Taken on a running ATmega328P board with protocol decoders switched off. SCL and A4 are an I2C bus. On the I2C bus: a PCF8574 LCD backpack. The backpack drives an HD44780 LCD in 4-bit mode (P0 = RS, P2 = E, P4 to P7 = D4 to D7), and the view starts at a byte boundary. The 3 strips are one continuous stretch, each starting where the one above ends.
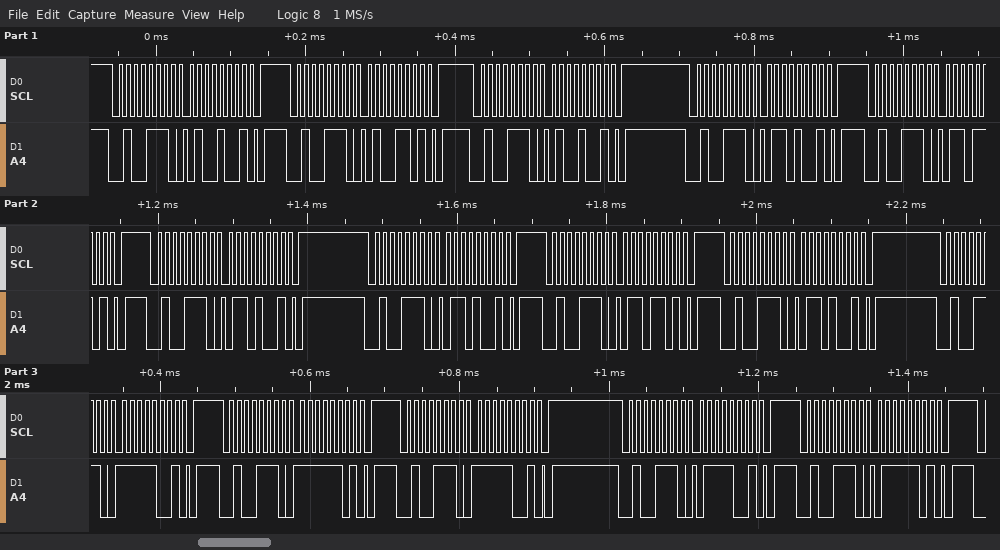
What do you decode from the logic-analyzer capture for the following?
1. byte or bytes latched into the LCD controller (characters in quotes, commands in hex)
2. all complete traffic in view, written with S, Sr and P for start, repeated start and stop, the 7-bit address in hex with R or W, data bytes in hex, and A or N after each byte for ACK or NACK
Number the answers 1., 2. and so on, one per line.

1. 'F' 'o'
2. S 27W A 49 A P S 27W A 4D A P S 27W A 49 A P S 27W A 69 A P S 27W A 6D A P S 27W A 69 A P S 27W A 69 A P S 27W A 6D A P S 27W A 69 A P S 27W A F9 A P S 27W A FD A P S 27W A F9 A P S 27W A 79 A P S 27W A 7D A P
